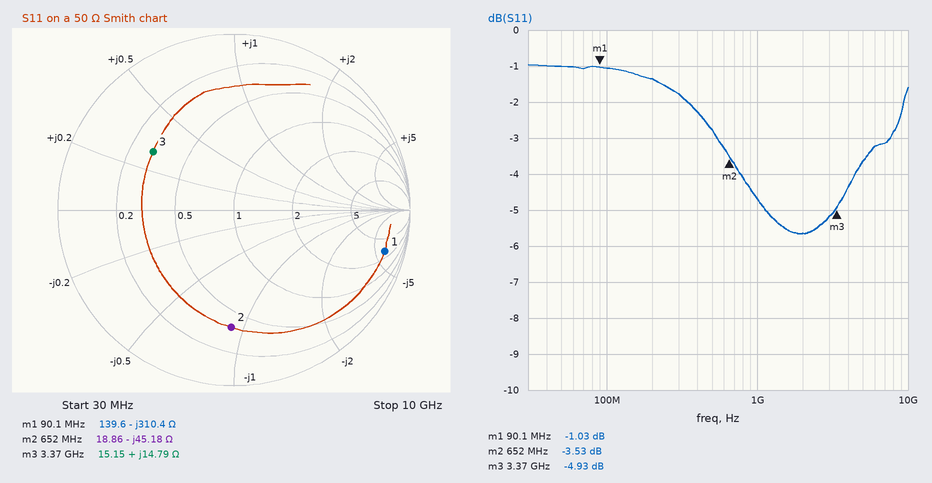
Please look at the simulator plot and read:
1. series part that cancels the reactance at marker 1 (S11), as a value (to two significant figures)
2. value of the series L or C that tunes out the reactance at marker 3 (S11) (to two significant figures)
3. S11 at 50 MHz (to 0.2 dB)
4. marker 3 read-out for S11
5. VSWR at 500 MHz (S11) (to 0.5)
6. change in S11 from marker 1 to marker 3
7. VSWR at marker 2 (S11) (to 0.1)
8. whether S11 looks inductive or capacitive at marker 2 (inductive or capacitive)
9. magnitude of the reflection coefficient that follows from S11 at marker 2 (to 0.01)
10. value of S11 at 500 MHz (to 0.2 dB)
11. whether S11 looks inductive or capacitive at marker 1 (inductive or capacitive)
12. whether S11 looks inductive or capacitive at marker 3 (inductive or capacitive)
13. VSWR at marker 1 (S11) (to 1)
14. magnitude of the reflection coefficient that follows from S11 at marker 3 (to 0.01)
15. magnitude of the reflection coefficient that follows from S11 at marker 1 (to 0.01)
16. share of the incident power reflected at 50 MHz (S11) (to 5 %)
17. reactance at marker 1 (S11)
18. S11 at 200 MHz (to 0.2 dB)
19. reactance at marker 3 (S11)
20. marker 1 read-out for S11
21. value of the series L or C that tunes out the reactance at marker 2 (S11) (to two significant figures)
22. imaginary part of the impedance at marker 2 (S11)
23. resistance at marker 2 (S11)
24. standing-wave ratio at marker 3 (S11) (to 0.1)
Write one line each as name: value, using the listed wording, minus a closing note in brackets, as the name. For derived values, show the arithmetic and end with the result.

series part that cancels the reactance at marker 1 (S11), as a value: L = 310.4 Ω/(2π × 90.1 MHz) ≈ 548 nH, so 550 nH to two significant figures
value of the series L or C that tunes out the reactance at marker 3 (S11): C = 1/(2π × 3.37 GHz × 14.79 Ω) ≈ 3.2 pF
S11 at 50 MHz: -1.0 dB
marker 3 read-out for S11: -4.93 dB
VSWR at 500 MHz (S11): |Γ| = 10^(-2.8/20) = 0.7244; VSWR = (1 + 0.7244)/(1 − 0.7244) ≈ 6.26, so 6.5 to the nearest 0.5
change in S11 from marker 1 to marker 3: -4.93 − (-1.03) = -3.90 dB
VSWR at marker 2 (S11): 5.0
whether S11 looks inductive or capacitive at marker 2: capacitive
magnitude of the reflection coefficient that follows from S11 at marker 2: 10^(-3.53/20) ≈ 0.67
value of S11 at 500 MHz: -2.8 dB
whether S11 looks inductive or capacitive at marker 1: capacitive
whether S11 looks inductive or capacitive at marker 3: inductive
VSWR at marker 1 (S11): 17
magnitude of the reflection coefficient that follows from S11 at marker 3: 10^(-4.93/20) ≈ 0.57
magnitude of the reflection coefficient that follows from S11 at marker 1: 10^(-1.03/20) ≈ 0.89
share of the incident power reflected at 50 MHz (S11): 10^(-1/10) ≈ 79.4 %, so 80 % to the nearest 5 %
reactance at marker 1: -310.4 Ω
S11 at 200 MHz: -1.4 dB
reactance at marker 3: +14.79 Ω
marker 1 read-out for S11: -1.03 dB
value of the series L or C that tunes out the reactance at marker 2 (S11): L = 45.18 Ω/(2π × 652 MHz) ≈ 11 nH
imaginary part of the impedance at marker 2: -45.18 Ω
resistance at marker 2: 18.86 Ω
standing-wave ratio at marker 3 (S11): 3.6
